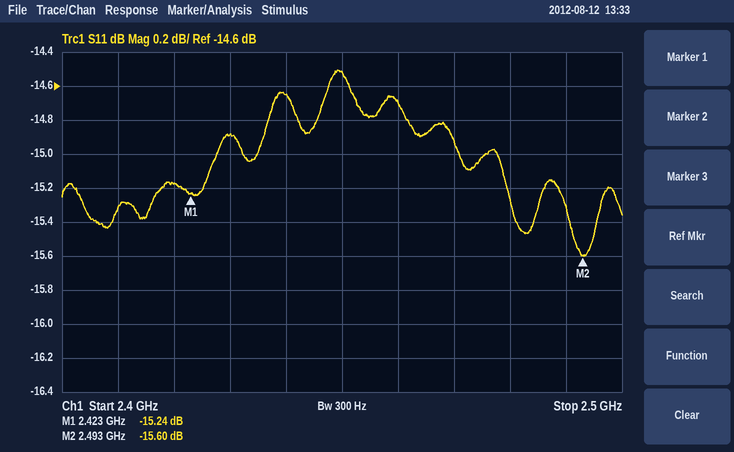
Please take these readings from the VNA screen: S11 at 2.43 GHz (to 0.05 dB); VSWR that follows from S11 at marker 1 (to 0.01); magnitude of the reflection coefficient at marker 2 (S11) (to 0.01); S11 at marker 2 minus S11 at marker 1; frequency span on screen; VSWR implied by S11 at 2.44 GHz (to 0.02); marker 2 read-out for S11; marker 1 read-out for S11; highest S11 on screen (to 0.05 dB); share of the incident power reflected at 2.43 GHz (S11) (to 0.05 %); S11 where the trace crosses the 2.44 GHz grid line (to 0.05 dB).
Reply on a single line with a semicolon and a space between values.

-14.90 dB; 1.42; 0.17; -0.36 dB; 100 MHz; 1.46; -15.60 dB; -15.24 dB; -14.50 dB; 3.25 %; -14.65 dB
